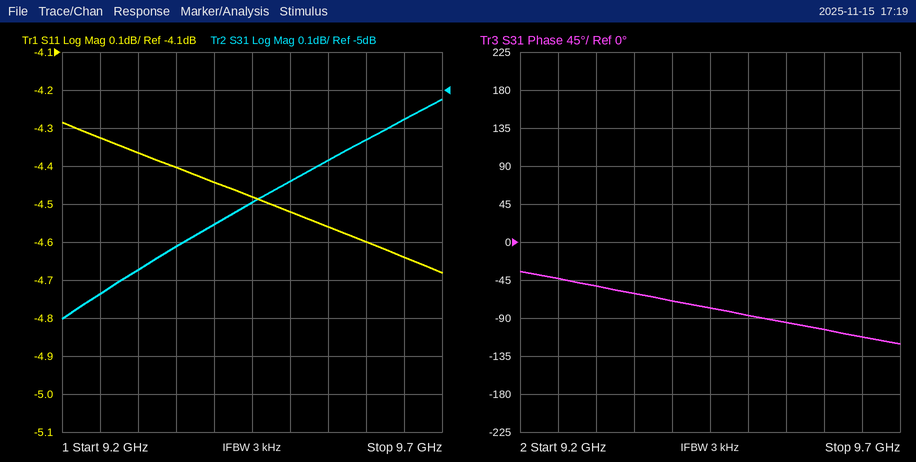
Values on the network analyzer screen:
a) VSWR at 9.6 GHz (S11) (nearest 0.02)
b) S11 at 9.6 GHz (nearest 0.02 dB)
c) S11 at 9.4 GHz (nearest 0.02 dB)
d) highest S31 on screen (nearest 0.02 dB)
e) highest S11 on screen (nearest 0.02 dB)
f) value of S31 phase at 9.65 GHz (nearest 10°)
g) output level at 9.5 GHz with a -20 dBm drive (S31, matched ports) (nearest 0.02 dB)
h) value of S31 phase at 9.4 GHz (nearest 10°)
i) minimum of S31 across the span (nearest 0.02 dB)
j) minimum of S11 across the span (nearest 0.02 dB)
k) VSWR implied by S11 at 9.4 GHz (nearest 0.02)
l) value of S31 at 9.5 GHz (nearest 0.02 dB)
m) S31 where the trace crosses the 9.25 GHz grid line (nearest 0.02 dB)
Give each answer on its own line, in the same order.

3.86
-4.60 dB
-4.44 dB
-5.02 dB
-4.28 dB
-110°
-25.24 dBm
-70°
-5.60 dB
-4.68 dB
4.00
-5.24 dB
-5.54 dB
